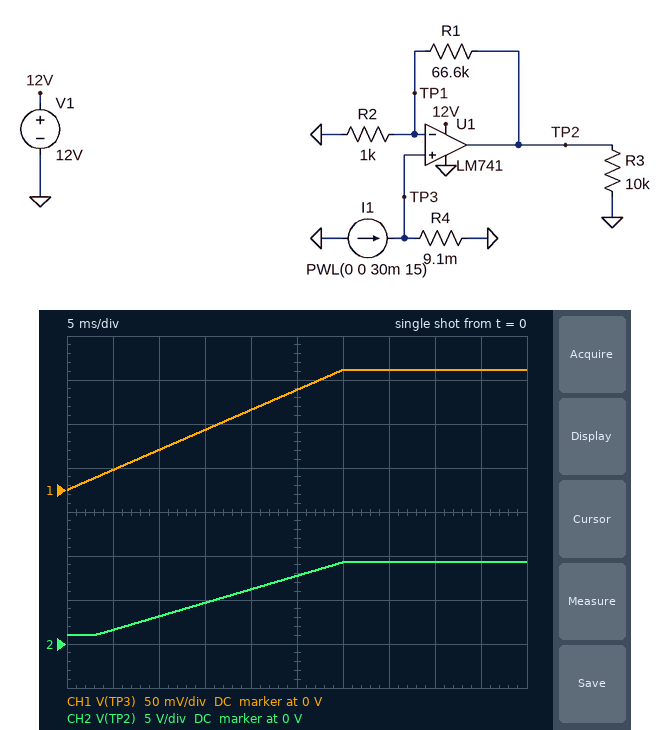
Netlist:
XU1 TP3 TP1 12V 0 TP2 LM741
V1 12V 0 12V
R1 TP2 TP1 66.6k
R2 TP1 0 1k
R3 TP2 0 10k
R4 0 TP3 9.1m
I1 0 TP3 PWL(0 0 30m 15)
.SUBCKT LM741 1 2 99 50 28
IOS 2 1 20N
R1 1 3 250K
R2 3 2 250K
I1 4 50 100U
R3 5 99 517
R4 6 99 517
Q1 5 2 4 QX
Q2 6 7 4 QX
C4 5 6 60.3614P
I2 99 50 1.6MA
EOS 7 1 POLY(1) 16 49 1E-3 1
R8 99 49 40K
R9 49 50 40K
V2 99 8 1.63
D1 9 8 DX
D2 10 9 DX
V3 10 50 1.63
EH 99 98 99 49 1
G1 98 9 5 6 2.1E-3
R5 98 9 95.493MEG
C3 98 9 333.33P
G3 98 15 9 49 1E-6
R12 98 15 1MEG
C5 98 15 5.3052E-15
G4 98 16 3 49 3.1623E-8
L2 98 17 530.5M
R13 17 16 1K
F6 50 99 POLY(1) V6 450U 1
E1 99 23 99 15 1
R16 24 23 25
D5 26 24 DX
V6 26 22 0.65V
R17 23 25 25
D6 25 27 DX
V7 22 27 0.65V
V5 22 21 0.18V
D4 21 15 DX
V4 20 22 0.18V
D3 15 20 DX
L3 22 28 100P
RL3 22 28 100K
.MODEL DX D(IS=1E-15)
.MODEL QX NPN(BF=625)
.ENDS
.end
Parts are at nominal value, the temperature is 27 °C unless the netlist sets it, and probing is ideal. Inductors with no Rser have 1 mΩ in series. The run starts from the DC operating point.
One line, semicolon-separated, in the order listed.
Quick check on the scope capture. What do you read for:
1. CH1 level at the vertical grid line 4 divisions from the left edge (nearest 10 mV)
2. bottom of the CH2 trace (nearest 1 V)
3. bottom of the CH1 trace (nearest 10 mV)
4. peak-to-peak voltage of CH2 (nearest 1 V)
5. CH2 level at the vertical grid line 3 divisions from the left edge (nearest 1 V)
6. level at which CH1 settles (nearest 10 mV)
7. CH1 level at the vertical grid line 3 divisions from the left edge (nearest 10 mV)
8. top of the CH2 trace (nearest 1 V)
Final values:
90 mV; 1 V; 0 V; 8 V; 5 V; 140 mV; 70 mV; 9 V
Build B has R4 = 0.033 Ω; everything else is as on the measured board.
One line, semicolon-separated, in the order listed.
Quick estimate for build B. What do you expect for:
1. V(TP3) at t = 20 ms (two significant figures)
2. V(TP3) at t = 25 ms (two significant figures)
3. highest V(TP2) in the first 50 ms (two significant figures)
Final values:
330 mV; 410 mV; 11 V
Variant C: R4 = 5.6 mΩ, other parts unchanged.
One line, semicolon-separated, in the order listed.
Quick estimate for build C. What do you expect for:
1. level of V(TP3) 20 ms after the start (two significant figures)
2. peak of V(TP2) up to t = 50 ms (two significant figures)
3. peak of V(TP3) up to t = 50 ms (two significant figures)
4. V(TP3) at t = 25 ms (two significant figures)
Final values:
56 mV; 5.7 V; 84 mV; 70 mV
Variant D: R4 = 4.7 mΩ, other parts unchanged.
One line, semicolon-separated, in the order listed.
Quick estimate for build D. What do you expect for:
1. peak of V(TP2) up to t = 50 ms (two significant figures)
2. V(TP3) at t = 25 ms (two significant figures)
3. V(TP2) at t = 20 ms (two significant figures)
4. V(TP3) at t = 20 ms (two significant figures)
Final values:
4.8 V; 59 mV; 3.2 V; 47 mV
